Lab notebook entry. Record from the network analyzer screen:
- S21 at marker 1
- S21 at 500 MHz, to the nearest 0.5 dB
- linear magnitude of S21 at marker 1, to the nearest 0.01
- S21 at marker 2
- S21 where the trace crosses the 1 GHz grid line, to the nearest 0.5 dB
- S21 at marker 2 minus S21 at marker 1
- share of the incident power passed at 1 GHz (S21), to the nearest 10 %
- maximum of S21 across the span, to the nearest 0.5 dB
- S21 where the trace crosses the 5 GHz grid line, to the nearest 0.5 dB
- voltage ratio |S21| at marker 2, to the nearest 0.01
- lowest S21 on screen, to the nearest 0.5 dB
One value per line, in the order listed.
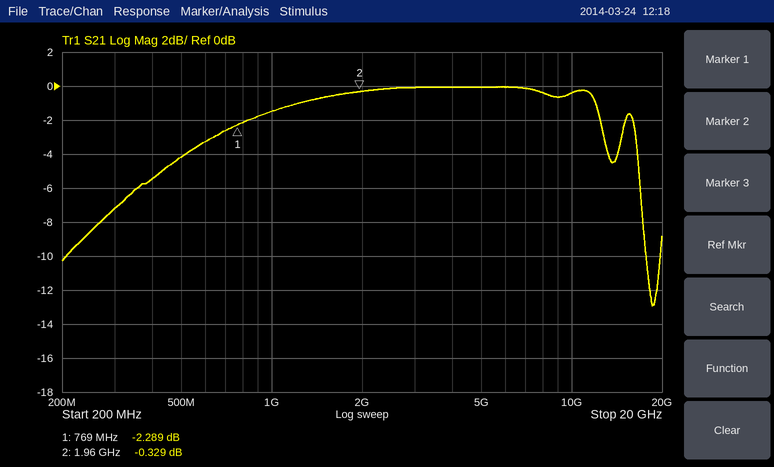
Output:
-2.289 dB
-4.0 dB
0.77
-0.329 dB
-1.5 dB
1.960 dB
70 %
0.0 dB
0.0 dB
0.96
-13.0 dB
